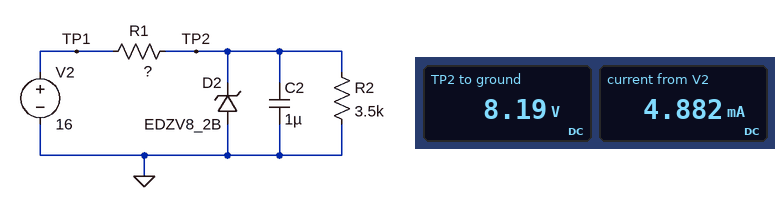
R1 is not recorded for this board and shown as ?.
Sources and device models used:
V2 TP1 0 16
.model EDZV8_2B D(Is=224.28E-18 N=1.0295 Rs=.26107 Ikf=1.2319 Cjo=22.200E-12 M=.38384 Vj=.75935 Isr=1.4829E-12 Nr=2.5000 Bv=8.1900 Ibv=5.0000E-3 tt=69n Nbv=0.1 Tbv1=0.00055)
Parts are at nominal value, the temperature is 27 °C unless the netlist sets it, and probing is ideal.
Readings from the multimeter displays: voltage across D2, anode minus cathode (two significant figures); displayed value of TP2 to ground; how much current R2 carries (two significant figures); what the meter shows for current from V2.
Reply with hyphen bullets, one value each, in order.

- -8.2 V
- 8.19 V
- 2.3 mA
- 4.882 mA
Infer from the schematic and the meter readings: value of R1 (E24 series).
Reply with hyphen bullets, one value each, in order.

- 1.6 kΩ
